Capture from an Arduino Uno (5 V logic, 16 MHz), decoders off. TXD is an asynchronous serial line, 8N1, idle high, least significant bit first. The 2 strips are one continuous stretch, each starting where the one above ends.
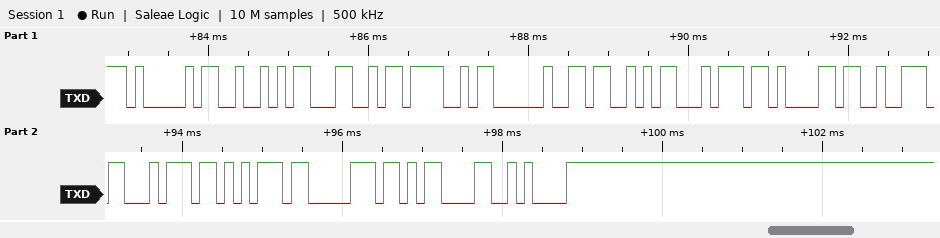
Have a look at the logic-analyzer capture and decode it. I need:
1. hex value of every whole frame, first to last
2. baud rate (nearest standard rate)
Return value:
0x41 0x52 0x4C 0x4F 0x20 0x53 0x74 0x61 0x72 0x74 0x75 0x70 0x0D 0x0A
9600 baud
